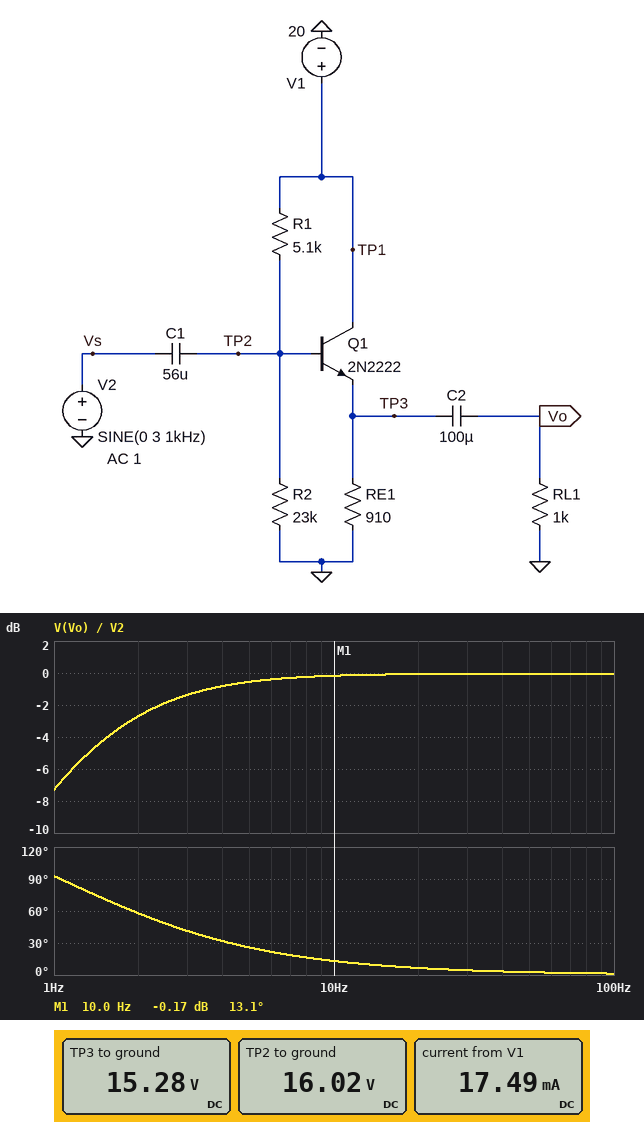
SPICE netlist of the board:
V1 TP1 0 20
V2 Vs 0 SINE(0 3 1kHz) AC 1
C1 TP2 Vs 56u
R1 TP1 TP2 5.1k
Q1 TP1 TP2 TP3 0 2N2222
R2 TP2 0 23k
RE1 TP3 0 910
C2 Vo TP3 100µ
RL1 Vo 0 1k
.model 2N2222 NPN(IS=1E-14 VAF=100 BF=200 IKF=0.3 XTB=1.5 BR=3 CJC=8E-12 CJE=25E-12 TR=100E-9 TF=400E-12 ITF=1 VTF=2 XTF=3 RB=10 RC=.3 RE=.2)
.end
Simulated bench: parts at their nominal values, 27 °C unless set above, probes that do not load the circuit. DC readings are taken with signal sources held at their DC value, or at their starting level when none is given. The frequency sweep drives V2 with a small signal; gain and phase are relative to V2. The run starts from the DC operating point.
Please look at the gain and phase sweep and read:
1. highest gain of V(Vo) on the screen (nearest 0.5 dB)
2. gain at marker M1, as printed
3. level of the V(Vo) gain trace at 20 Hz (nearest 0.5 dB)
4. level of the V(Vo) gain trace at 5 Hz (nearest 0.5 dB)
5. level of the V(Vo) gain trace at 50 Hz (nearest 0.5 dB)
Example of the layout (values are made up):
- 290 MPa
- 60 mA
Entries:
- 0 dB
- -0.17 dB
- 0 dB
- -0.5 dB
- 0 dB
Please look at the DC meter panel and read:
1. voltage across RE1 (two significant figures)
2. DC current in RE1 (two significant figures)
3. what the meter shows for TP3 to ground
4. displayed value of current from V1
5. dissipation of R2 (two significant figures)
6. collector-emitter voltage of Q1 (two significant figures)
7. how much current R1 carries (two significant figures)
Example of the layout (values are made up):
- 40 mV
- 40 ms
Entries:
- 15 V
- 17 mA
- 15.28 V
- 17.49 mA
- 11 mW
- 4.7 V
- 780 µA
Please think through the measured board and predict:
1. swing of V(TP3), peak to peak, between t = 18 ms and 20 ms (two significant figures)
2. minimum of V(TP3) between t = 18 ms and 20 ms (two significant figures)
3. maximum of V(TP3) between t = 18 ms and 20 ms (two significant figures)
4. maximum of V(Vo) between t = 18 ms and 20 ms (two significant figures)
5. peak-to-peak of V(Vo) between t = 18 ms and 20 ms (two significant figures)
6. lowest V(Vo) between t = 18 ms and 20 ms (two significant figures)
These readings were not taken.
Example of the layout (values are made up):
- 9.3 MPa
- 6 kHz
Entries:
- 6.0 V
- 12 V
- 18 V
- 3.0 V
- 6.0 V
- -3.0 V
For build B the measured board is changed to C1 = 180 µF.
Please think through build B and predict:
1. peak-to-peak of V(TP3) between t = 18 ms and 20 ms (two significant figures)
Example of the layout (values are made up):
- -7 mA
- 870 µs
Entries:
- 6.0 V
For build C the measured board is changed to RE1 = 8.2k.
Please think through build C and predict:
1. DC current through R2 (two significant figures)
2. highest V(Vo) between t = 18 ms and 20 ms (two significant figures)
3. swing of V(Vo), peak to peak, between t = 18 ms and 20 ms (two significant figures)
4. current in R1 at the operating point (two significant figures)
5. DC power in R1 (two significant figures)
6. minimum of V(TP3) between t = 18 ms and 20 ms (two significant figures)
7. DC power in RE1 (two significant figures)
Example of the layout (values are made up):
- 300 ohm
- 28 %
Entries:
- 710 µA
- 2.9 V
- 4.6 V
- 720 µA
- 2.6 mW
- 14 V
- 30 mW
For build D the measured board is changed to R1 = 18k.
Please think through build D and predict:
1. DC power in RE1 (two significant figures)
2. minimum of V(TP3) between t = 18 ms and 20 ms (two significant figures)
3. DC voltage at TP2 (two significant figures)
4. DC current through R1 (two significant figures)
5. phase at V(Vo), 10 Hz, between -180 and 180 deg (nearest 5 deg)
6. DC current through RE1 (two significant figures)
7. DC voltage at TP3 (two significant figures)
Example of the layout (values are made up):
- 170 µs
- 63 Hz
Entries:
- 110 mW
- 7.0 V
- 11 V
- 520 µA
- 10 deg
- 11 mA
- 10 V
